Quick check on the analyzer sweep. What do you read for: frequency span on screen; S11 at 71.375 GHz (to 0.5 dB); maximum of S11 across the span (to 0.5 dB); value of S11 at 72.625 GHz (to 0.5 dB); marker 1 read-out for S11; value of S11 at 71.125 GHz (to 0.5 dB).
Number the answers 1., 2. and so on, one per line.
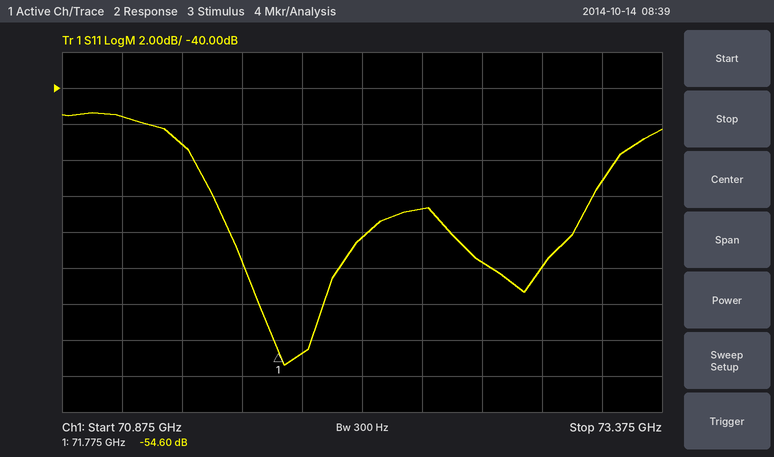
1. 2.5 GHz
2. -43.0 dB
3. -41.5 dB
4. -49.5 dB
5. -54.60 dB
6. -41.5 dB
